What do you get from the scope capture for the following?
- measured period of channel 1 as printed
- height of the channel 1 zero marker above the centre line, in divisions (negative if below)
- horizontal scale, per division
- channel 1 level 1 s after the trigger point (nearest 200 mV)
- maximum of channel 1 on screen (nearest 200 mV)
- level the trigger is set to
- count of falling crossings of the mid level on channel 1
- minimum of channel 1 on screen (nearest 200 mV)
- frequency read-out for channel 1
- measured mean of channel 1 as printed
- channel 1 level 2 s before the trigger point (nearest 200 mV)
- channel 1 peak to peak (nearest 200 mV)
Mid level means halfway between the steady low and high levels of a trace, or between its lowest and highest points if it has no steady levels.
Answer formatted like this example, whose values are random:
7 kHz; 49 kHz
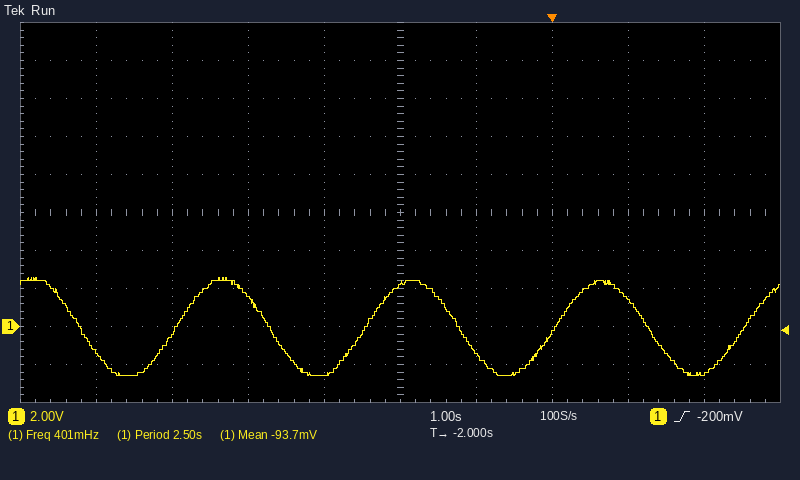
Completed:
2.50 s; -3.0 div; 1 s; 1.4 V; 2.6 V; -200 mV; 4; -2.6 V; 401 mHz; -93.7 mV; 2.2 V; 5.2 V
